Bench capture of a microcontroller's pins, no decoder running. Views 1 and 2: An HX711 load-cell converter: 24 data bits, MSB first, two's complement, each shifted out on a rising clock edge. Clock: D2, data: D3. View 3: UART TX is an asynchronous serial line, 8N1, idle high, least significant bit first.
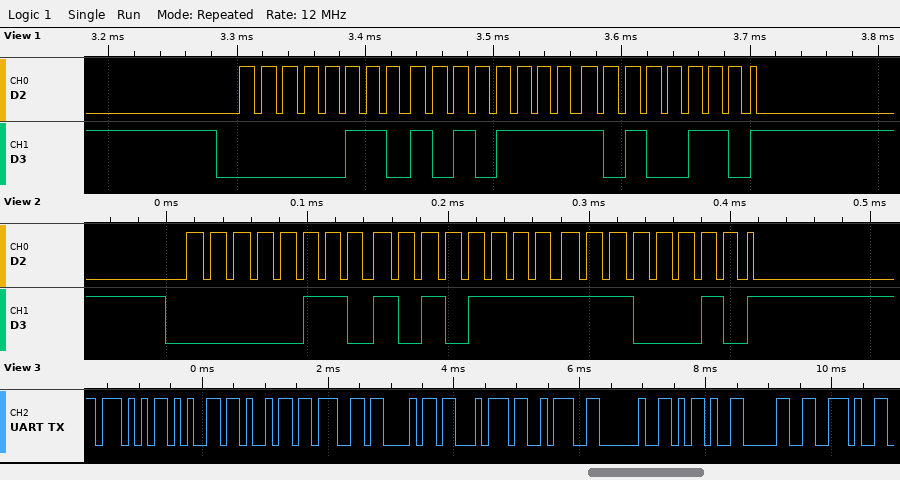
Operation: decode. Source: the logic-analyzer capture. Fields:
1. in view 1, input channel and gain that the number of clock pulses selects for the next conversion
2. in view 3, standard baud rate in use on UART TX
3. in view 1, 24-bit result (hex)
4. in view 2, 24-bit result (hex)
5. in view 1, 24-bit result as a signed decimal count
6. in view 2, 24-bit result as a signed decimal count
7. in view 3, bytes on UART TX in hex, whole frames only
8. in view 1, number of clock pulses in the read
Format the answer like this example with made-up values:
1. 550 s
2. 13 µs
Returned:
1. channel A, gain 128
2. 9600 baud
3. 0x06AFA6
4. 0x06AFE2
5. 438182
6. 438242
7. 0x57 0x65 0x69 0x67 0x68 0x74 0x3A 0x20 0x2D 0x30 0x2E
8. 25
